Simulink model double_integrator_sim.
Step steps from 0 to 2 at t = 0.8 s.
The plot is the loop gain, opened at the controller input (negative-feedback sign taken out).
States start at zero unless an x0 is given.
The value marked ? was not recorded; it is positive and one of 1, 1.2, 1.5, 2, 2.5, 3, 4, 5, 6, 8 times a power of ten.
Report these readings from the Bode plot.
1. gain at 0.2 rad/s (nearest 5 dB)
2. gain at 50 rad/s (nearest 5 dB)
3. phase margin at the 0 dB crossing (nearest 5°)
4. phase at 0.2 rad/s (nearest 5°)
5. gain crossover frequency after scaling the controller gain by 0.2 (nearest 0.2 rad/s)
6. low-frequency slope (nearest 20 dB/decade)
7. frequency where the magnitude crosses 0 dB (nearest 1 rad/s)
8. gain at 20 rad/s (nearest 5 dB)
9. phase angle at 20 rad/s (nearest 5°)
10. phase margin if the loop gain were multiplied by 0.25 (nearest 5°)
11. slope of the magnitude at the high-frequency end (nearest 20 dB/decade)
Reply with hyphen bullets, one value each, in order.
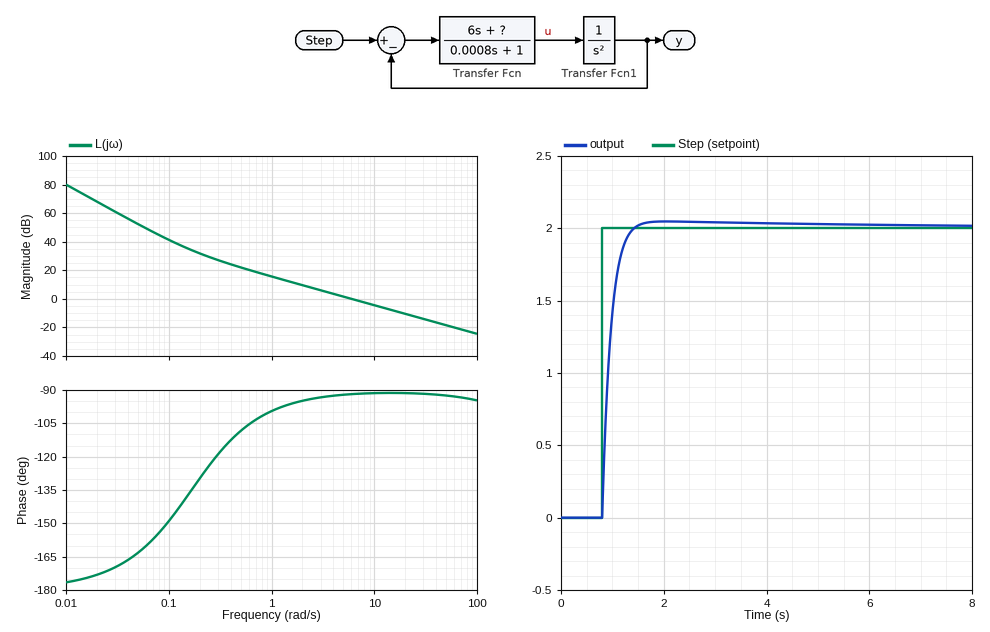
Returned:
- 30 dB
- -20 dB
- 90°
- -130°
- 1.2 rad/s
- -40 dB/decade
- 6 rad/s
- -10 dB
- -90°
- 85°
- -20 dB/decade
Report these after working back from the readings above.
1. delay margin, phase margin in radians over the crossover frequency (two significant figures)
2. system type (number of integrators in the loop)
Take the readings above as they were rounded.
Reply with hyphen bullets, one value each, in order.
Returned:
- 0.26 s
- 2
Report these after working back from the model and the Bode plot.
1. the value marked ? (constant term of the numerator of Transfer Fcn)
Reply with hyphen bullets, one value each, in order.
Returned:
- 1
